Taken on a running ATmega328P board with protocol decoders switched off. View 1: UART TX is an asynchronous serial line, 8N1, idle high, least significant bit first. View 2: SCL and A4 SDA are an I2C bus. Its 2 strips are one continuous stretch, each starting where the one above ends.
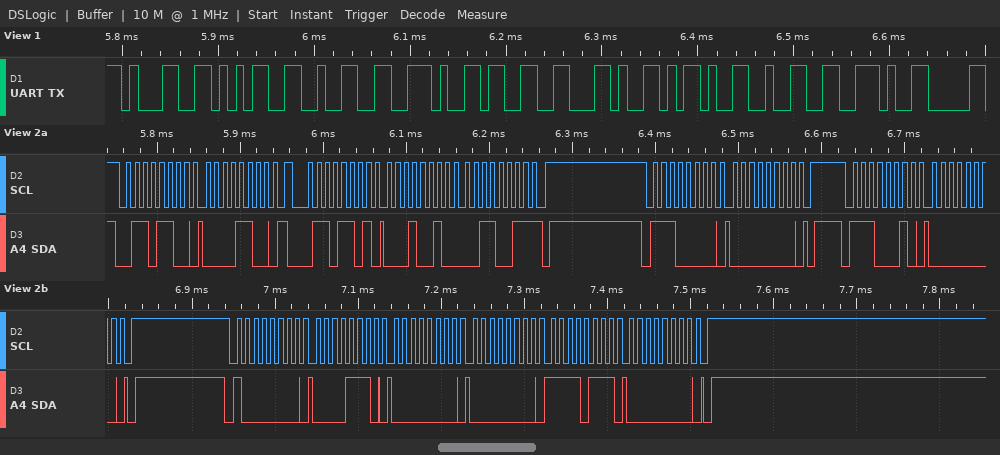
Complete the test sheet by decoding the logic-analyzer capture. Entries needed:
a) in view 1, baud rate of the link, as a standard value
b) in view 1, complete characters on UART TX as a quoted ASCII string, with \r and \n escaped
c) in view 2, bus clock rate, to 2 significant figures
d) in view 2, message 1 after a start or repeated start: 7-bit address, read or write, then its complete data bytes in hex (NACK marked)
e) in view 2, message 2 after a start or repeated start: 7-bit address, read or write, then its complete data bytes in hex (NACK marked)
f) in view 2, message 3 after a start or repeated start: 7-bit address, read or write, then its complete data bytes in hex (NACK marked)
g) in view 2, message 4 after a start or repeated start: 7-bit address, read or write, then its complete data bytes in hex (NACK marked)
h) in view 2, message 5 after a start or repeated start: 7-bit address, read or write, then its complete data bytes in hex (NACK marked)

115200 baud
"152.3,-2."
100 kHz
0x36 write: 0C
0x36 read: 12 33 NACK
0x70 write: 00
0x71 write: 00
0x40 write: 0E 00 00 F7 00
